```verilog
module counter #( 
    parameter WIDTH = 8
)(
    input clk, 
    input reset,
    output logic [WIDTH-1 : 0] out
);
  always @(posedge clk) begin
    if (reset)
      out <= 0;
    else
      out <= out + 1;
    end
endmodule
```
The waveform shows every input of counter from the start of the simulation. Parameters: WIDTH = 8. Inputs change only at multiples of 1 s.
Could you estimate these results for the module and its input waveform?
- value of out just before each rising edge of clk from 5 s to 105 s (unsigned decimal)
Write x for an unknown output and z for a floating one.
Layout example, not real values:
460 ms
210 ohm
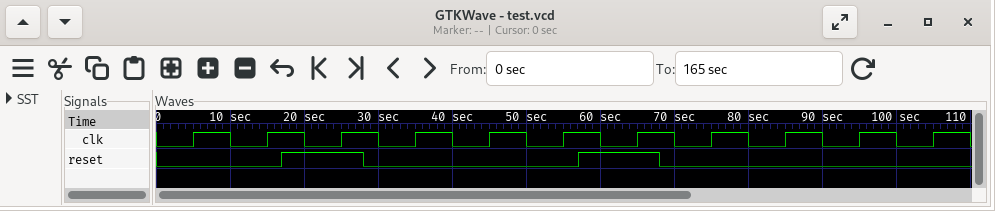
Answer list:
x, x, x, 0, 1, 2, 3, 0, 1, 2, 3
